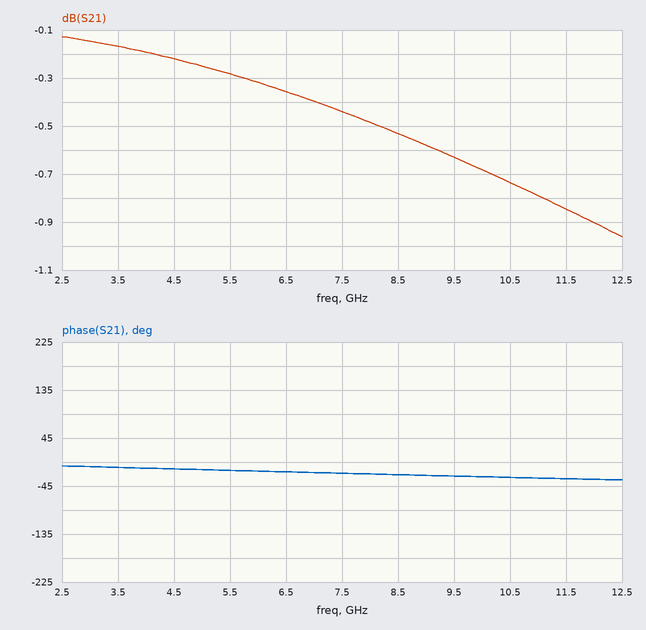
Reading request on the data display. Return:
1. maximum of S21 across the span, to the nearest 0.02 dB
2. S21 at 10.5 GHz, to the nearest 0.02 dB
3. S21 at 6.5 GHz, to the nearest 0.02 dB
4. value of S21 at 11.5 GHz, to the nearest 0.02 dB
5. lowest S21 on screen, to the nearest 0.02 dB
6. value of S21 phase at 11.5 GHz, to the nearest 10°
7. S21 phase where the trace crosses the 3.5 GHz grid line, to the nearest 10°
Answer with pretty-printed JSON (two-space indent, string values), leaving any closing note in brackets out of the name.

{
  "maximum of S21 across the span, to the nearest 0.02 dB": "-0.12 dB",
  "S21 at 10.5 GHz, to the nearest 0.02 dB": "-0.74 dB",
  "S21 at 6.5 GHz, to the nearest 0.02 dB": "-0.36 dB",
  "value of S21 at 11.5 GHz, to the nearest 0.02 dB": "-0.84 dB",
  "lowest S21 on screen, to the nearest 0.02 dB": "-0.96 dB",
  "value of S21 phase at 11.5 GHz, to the nearest 10°": "-30°",
  "S21 phase where the trace crosses the 3.5 GHz grid line, to the nearest 10°": "-10°"
}
